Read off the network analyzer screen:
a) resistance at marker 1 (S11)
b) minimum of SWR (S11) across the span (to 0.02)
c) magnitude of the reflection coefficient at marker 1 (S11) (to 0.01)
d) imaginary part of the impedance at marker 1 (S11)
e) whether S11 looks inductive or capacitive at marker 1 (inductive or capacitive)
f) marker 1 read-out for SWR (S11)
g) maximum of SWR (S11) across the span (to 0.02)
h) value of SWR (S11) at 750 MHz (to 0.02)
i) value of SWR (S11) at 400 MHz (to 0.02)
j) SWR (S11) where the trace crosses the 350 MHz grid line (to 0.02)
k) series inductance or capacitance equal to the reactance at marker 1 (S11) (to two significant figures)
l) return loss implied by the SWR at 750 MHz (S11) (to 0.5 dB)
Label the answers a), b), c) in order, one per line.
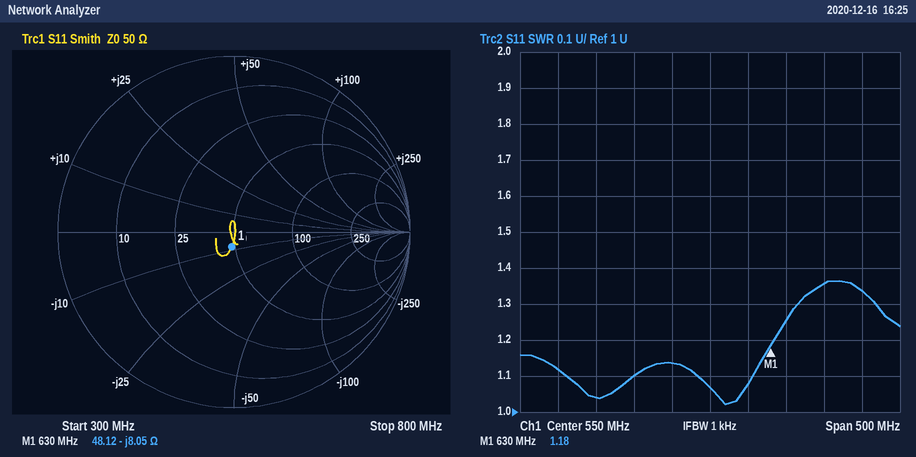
a) 48.12 Ω
b) 1.02
c) 0.08
d) -8.05 Ω
e) capacitive
f) 1.18
g) 1.36
h) 1.34
i) 1.04
j) 1.12
k) 31 pF
l) 17.0 dB
